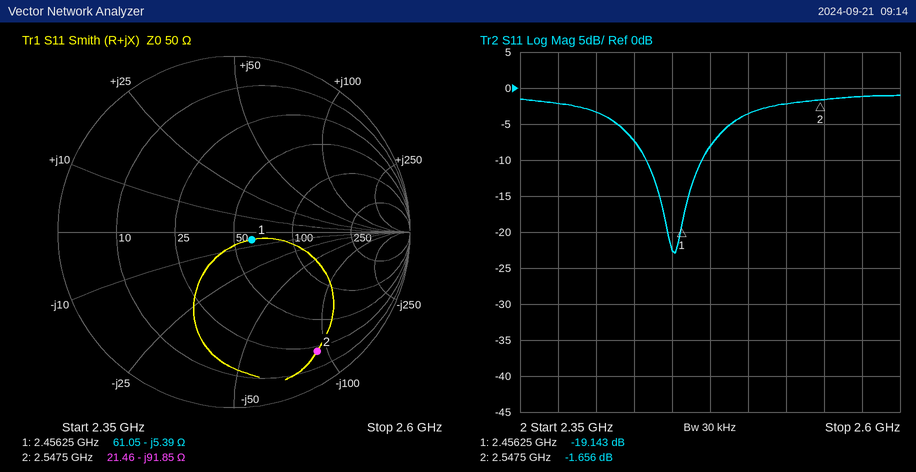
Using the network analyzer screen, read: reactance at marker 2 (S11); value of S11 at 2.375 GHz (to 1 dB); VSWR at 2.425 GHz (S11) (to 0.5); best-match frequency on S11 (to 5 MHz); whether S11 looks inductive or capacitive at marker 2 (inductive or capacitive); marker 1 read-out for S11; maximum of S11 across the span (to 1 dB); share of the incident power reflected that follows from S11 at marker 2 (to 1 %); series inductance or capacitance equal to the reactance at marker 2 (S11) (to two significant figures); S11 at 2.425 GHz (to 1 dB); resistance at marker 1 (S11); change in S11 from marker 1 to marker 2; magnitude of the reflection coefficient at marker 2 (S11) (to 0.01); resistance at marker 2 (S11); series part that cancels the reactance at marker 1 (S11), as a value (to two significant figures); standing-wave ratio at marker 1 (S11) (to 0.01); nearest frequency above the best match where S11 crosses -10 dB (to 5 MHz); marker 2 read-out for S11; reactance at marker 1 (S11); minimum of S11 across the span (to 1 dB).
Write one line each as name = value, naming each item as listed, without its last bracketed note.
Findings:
reactance at marker 2 = -91.85 Ω
value of S11 at 2.375 GHz = -2 dB
VSWR at 2.425 GHz (S11) = 2.5
best-match frequency on S11 = 2.450 GHz
whether S11 looks inductive or capacitive at marker 2 = capacitive
marker 1 read-out for S11 = -19.143 dB
maximum of S11 across the span = -1 dB
share of the incident power reflected that follows from S11 at marker 2 = 68 %
series inductance or capacitance equal to the reactance at marker 2 (S11) = 680 fF
S11 at 2.425 GHz = -7 dB
resistance at marker 1 = 61.05 Ω
change in S11 from marker 1 to marker 2 = 17.487 dB
magnitude of the reflection coefficient at marker 2 (S11) = 0.83
resistance at marker 2 = 21.46 Ω
series part that cancels the reactance at marker 1 (S11), as a value = 350 pH
standing-wave ratio at marker 1 (S11) = 1.25
nearest frequency above the best match where S11 crosses -10 dB = 2.470 GHz
marker 2 read-out for S11 = -1.656 dB
reactance at marker 1 = -5.39 Ω
minimum of S11 across the span = -23 dB
